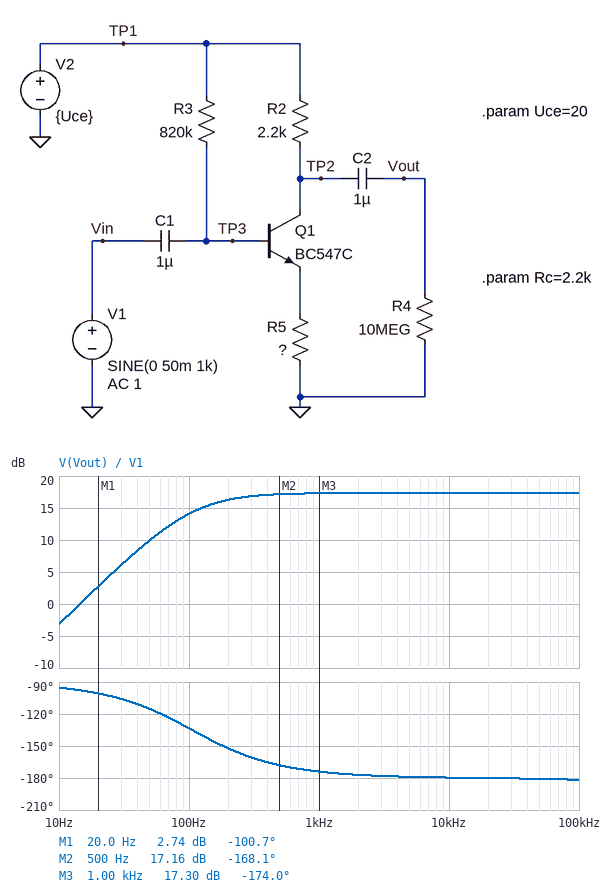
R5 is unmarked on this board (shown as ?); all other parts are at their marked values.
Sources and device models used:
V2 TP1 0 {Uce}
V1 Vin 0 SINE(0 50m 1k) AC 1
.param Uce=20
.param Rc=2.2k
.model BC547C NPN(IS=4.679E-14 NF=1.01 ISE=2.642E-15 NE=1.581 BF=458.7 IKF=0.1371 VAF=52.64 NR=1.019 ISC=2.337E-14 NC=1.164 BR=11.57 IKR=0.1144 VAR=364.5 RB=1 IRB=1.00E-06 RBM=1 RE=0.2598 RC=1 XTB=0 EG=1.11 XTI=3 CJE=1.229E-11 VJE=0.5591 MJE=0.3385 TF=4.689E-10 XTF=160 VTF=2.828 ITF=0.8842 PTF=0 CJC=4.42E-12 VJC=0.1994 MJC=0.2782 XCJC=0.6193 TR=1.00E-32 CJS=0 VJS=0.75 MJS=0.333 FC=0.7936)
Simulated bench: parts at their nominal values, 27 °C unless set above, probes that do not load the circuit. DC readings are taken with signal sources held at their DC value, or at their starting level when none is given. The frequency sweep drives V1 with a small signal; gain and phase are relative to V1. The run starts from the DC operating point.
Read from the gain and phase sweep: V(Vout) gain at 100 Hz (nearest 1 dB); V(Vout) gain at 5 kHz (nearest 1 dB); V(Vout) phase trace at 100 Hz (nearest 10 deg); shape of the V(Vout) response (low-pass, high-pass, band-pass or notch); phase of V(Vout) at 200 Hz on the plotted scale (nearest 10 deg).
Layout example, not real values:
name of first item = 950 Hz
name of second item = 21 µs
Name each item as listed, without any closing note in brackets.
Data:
V(Vout) gain at 100 Hz = 14 dB
V(Vout) gain at 5 kHz = 17 dB
V(Vout) phase trace at 100 Hz = -130 deg
shape of the V(Vout) response = high-pass
phase of V(Vout) at 200 Hz on the plotted scale = -150 deg
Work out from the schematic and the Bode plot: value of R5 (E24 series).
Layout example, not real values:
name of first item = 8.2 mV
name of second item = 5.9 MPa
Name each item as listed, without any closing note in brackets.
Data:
value of R5 = 240 Ω
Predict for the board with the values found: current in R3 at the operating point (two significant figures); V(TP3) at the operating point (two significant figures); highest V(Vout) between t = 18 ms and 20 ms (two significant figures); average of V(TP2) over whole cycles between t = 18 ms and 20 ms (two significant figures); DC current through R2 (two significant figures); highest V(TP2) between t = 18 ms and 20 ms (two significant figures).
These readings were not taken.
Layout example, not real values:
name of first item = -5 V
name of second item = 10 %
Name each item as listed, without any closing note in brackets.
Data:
current in R3 at the operating point = 21 µA
V(TP3) at the operating point = 2.6 V
highest V(Vout) between t = 18 ms and 20 ms = 790 mV
average of V(TP2) over whole cycles between t = 18 ms and 20 ms = 2.5 V
DC current through R2 = 8.1 mA
highest V(TP2) between t = 18 ms and 20 ms = 2.9 V
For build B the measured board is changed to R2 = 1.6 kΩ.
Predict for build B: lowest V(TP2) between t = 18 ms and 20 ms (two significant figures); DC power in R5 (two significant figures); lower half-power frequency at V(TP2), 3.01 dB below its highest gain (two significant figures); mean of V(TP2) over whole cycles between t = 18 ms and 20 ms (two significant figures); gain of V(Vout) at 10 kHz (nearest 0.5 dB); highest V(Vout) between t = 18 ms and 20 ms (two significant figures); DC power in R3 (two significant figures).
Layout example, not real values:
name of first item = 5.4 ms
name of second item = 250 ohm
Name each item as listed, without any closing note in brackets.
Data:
lowest V(TP2) between t = 18 ms and 20 ms = 4.8 V
DC power in R5 = 21 mW
lower half-power frequency at V(TP2), 3.01 dB below its highest gain = 2.2 Hz
mean of V(TP2) over whole cycles between t = 18 ms and 20 ms = 5.1 V
gain of V(Vout) at 10 kHz = 16.5 dB
highest V(Vout) between t = 18 ms and 20 ms = 330 mV
DC power in R3 = 360 µW
